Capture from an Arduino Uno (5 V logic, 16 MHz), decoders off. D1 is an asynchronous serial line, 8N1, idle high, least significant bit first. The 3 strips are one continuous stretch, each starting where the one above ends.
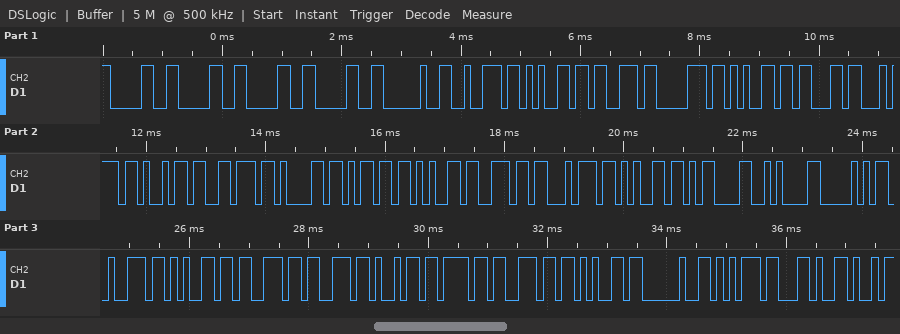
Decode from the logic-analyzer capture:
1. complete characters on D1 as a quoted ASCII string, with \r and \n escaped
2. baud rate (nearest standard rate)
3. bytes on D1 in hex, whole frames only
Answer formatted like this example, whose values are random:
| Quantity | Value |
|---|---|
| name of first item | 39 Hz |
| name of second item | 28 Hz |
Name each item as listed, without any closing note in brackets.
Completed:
| Quantity | Value |
|---|---|
| complete characters on D1 as a quoted ASCII string, with \r and \n escaped | "0000 respectivamente\r\nPressione u," |
| baud rate | 9600 baud |
| bytes on D1 in hex, whole frames only | 30 30 30 30 20 72 65 73 70 65 63 74 69 76 61 6D 65 6E 74 65 0D 0A 50 72 65 73 73 69 6F 6E 65 20 75 2C |
